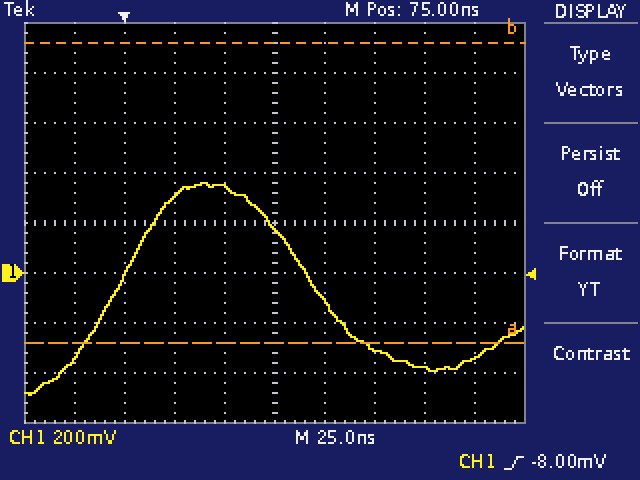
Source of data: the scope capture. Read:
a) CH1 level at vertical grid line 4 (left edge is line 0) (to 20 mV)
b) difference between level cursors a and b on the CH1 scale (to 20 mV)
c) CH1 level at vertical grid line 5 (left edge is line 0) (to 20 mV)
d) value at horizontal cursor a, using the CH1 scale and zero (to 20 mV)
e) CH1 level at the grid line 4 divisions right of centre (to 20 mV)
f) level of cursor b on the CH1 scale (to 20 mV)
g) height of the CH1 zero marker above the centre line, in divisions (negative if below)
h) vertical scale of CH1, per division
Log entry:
340 mV
1.20 V
180 mV
-280 mV
-340 mV
920 mV
-1.0 div
200 mV
